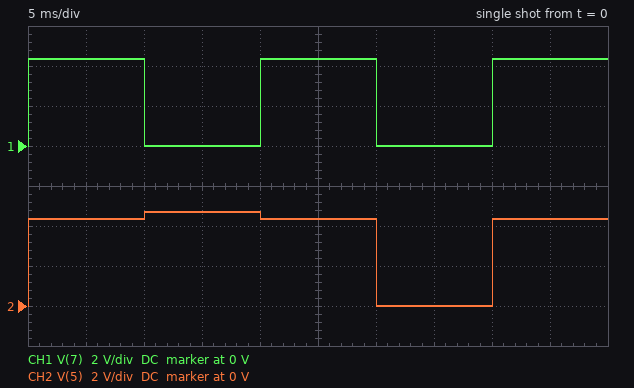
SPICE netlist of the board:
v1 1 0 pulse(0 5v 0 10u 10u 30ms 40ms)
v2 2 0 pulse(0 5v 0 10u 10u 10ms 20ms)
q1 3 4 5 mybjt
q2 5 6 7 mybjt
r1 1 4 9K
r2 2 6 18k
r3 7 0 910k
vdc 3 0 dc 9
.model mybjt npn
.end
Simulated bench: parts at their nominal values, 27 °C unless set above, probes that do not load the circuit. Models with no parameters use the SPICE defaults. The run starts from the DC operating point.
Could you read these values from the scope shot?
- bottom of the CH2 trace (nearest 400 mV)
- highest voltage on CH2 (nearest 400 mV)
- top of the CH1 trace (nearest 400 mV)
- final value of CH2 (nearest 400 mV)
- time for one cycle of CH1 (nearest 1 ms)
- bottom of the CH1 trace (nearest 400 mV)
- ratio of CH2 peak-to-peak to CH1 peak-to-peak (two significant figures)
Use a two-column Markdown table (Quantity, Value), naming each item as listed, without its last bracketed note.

| Quantity | Value |
|---|---|
| bottom of the CH2 trace | 0 V |
| highest voltage on CH2 | 4.8 V |
| top of the CH1 trace | 4.4 V |
| final value of CH2 | 4.4 V |
| time for one cycle of CH1 | 20 ms |
| bottom of the CH1 trace | 0 V |
| ratio of CH2 peak-to-peak to CH1 peak-to-peak | 1.1 |
